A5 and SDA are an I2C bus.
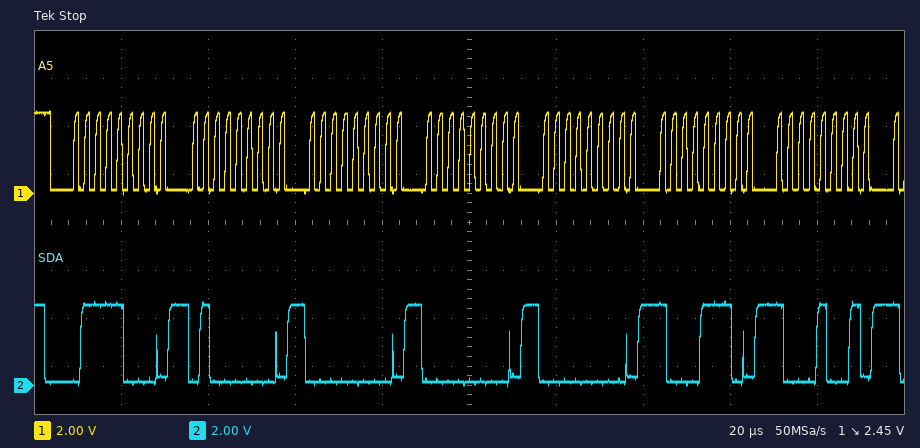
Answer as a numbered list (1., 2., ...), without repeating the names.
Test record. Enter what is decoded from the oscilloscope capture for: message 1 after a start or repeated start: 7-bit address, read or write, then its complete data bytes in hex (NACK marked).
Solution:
1. 0x3C write: 40 00 00 00 8E 89
